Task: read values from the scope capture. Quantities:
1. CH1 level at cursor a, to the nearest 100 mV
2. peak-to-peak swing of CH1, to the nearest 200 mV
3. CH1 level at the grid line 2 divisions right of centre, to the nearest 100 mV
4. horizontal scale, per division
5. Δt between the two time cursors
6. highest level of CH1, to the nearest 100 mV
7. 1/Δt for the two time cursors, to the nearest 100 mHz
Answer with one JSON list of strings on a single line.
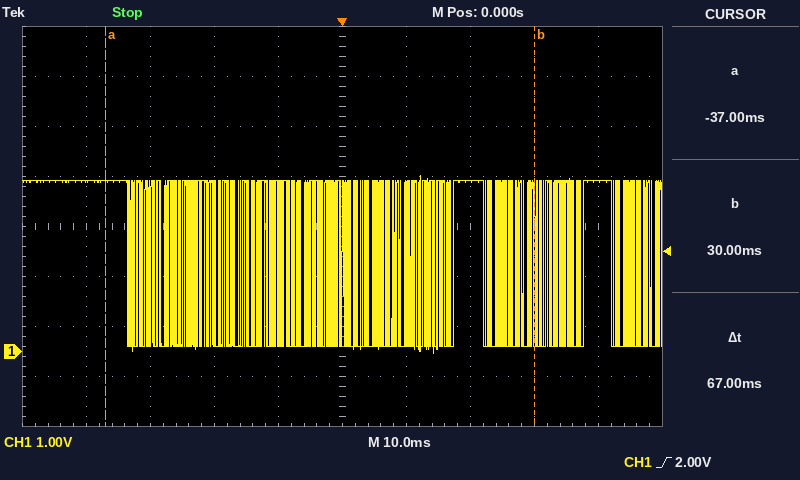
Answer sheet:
["3.4 V", "3.6 V", "3.4 V", "10 ms", "67 ms", "3.5 V", "14.9 Hz"]
